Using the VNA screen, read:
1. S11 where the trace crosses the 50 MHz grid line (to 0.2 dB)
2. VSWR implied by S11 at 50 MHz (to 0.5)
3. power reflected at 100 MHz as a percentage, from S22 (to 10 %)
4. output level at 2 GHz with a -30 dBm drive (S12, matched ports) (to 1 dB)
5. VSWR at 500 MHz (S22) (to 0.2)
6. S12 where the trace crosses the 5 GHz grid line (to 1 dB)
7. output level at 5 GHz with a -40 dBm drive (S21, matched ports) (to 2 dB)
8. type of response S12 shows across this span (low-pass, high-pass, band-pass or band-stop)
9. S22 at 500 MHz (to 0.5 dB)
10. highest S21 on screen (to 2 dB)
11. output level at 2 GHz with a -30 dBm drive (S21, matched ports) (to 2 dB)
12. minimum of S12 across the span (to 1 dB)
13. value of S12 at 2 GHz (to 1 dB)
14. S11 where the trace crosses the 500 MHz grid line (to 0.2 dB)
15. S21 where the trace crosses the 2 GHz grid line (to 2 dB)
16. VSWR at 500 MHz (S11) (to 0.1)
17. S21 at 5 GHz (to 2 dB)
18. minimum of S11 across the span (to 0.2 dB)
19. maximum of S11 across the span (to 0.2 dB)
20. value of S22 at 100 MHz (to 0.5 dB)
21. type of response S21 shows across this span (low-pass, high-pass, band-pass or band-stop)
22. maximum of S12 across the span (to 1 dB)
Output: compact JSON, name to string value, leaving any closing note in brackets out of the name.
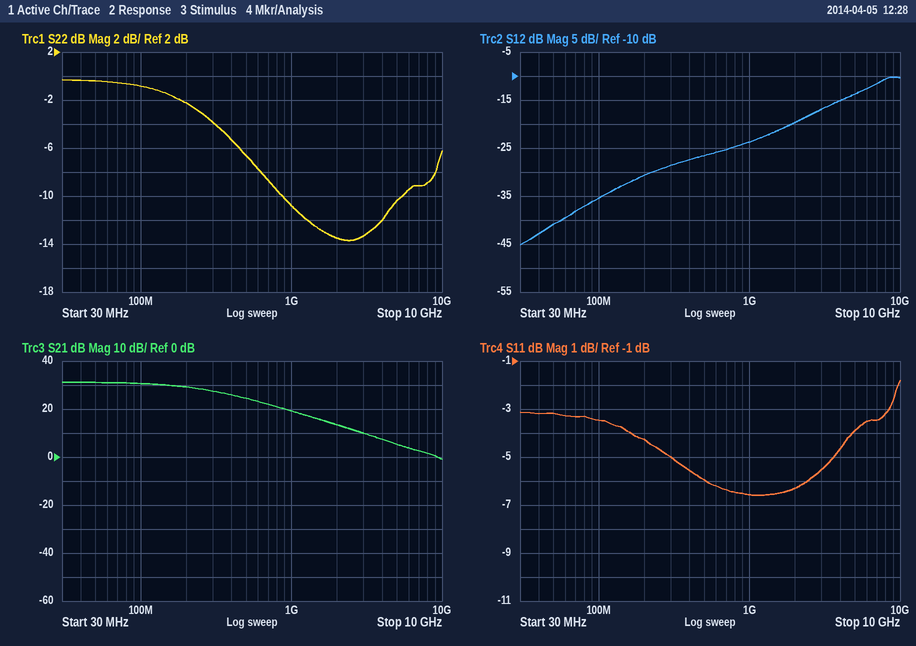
{"S11 where the trace crosses the 50 MHz grid line": "-3.2 dB", "VSWR implied by S11 at 50 MHz": "5.5", "power reflected at 100 MHz as a percentage, from S22": "80 %", "output level at 2 GHz with a -30 dBm drive (S12, matched ports)": "-50 dBm", "VSWR at 500 MHz (S22)": "2.8", "S12 where the trace crosses the 5 GHz grid line": "-14 dB", "output level at 5 GHz with a -40 dBm drive (S21, matched ports)": "-34 dBm", "type of response S12 shows across this span": "high-pass", "S22 at 500 MHz": "-6.5 dB", "highest S21 on screen": "32 dB", "output level at 2 GHz with a -30 dBm drive (S21, matched ports)": "-16 dBm", "minimum of S12 across the span": "-45 dB", "value of S12 at 2 GHz": "-20 dB", "S11 where the trace crosses the 500 MHz grid line": "-6.0 dB", "S21 where the trace crosses the 2 GHz grid line": "14 dB", "VSWR at 500 MHz (S11)": "3.0", "S21 at 5 GHz": "6 dB", "minimum of S11 across the span": "-6.6 dB", "maximum of S11 across the span": "-1.8 dB", "value of S22 at 100 MHz": "-1.0 dB", "type of response S21 shows across this span": "low-pass", "maximum of S12 across the span": "-10 dB"}
